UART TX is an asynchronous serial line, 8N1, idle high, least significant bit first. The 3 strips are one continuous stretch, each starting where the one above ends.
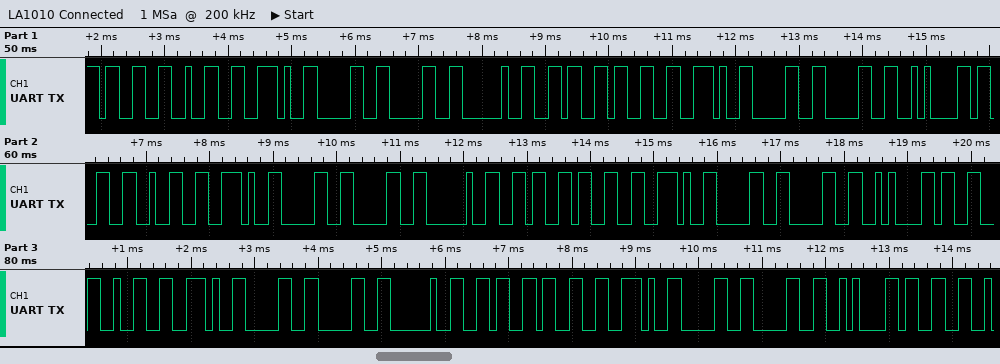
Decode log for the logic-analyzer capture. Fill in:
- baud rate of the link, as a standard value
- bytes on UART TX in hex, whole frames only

9600 baud
0x33 0x32 0x2E 0x30 0x30 0x20 0x36 0x33 0x2E 0x30 0x30 0x0A 0x33 0x32 0x2E 0x30 0x30 0x20 0x36 0x33 0x2E 0x30 0x30 0x0A 0x33 0x32 0x2E 0x30 0x30 0x20 0x36 0x33 0x2E 0x30 0x30 0x0A 0x33
